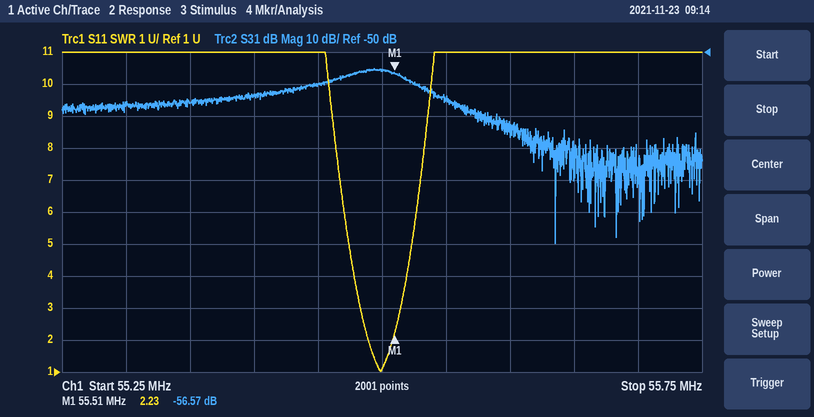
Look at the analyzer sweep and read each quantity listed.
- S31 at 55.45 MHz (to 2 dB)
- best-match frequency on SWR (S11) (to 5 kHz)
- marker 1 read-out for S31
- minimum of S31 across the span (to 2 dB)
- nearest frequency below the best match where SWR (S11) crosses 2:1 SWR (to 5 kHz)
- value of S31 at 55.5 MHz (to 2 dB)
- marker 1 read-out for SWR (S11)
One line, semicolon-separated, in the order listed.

-60 dB; 55.500 MHz; -56.57 dB; -110 dB; 55.490 MHz; -56 dB; 2.23
